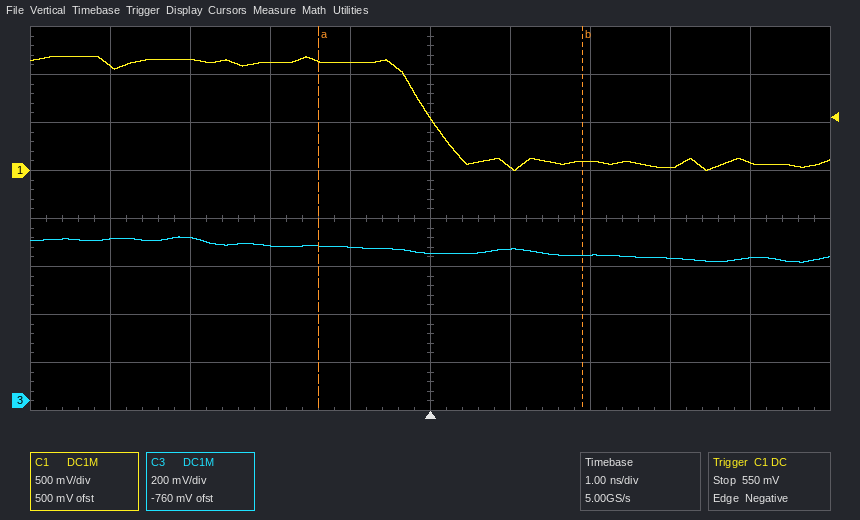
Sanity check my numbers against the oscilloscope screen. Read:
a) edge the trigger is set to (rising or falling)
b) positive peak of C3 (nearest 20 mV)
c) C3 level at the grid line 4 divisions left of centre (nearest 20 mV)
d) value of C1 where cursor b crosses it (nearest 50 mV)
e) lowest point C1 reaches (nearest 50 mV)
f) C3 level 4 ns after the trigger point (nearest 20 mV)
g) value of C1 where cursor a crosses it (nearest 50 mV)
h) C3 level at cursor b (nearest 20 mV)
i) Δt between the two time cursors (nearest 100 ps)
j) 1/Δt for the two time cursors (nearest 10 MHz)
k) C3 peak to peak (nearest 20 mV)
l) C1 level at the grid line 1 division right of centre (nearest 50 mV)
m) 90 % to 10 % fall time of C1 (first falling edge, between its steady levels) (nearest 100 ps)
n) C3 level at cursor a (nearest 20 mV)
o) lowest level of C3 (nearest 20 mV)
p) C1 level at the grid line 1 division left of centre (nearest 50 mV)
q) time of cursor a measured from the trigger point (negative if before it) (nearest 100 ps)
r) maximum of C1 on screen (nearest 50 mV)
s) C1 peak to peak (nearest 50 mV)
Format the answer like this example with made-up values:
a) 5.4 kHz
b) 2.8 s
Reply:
a) falling
b) 680 mV
c) 680 mV
d) 100 mV
e) 0 mV
f) 600 mV
g) 1.15 V
h) 600 mV
i) 3.3 ns
j) 300 MHz
k) 100 mV
l) 50 mV
m) 700 ps
n) 640 mV
o) 580 mV
p) 1.10 V
q) -1.4 ns
r) 1.20 V
s) 1.20 V
